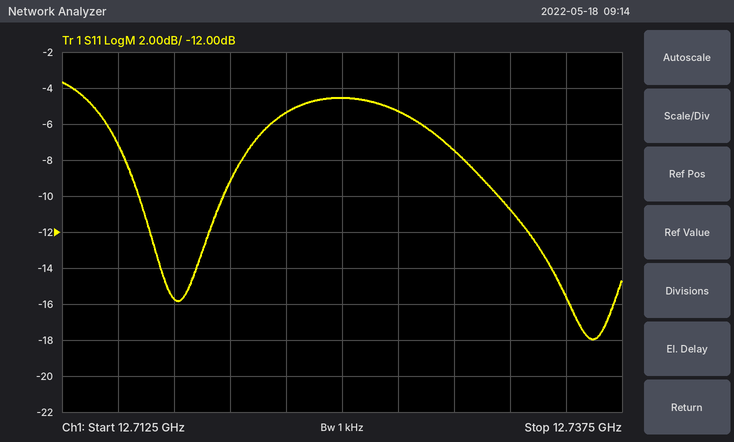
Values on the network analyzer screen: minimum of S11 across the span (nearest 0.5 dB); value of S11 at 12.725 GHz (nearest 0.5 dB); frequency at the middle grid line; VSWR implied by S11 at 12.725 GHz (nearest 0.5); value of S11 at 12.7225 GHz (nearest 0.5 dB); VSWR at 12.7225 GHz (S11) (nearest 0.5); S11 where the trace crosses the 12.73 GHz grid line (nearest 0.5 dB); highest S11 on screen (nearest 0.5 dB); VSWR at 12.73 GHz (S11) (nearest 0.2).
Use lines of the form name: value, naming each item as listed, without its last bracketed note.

minimum of S11 across the span: -18.0 dB
value of S11 at 12.725 GHz: -4.5 dB
frequency at the middle grid line: 12.725 GHz
VSWR implied by S11 at 12.725 GHz: 4.0
value of S11 at 12.7225 GHz: -5.5 dB
VSWR at 12.7225 GHz (S11): 3.5
S11 where the trace crosses the 12.73 GHz grid line: -7.5 dB
highest S11 on screen: -3.5 dB
VSWR at 12.73 GHz (S11): 2.4
